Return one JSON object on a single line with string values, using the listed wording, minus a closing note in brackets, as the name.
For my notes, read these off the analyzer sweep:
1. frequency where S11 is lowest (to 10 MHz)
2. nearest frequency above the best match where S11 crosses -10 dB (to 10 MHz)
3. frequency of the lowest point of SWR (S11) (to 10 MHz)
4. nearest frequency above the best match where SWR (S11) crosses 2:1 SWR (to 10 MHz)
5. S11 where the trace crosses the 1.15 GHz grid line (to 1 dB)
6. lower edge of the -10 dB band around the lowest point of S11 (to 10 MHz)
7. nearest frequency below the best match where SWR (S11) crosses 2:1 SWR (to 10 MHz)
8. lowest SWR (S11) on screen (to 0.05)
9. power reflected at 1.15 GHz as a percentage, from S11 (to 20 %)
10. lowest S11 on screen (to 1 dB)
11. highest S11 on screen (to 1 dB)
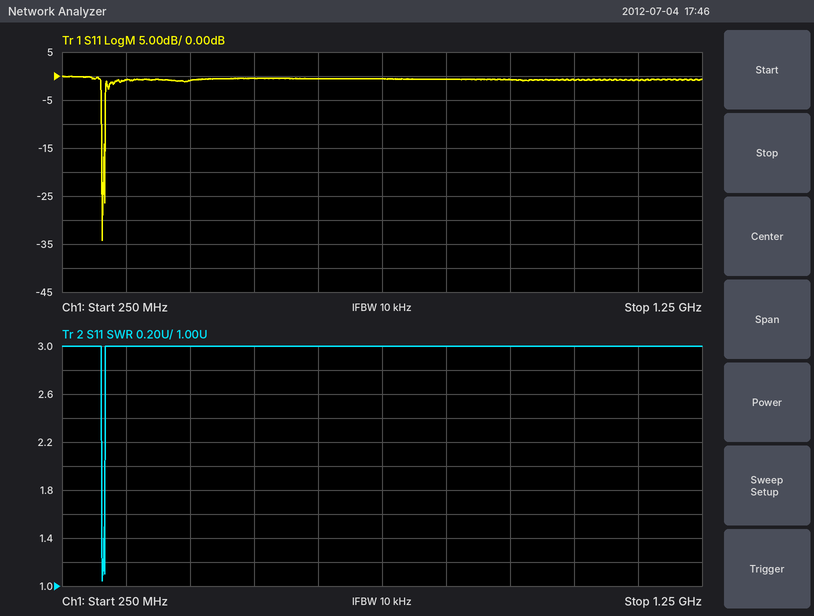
{"frequency where S11 is lowest": "310 MHz", "nearest frequency above the best match where S11 crosses -10 dB": "320 MHz", "frequency of the lowest point of SWR (S11)": "310 MHz", "nearest frequency above the best match where SWR (S11) crosses 2:1 SWR": "320 MHz", "S11 where the trace crosses the 1.15 GHz grid line": "-1 dB", "lower edge of the -10 dB band around the lowest point of S11": "310 MHz", "nearest frequency below the best match where SWR (S11) crosses 2:1 SWR": "310 MHz", "lowest SWR (S11) on screen": "1.05", "power reflected at 1.15 GHz as a percentage, from S11": "80 %", "lowest S11 on screen": "-34 dB", "highest S11 on screen": "0 dB"}
